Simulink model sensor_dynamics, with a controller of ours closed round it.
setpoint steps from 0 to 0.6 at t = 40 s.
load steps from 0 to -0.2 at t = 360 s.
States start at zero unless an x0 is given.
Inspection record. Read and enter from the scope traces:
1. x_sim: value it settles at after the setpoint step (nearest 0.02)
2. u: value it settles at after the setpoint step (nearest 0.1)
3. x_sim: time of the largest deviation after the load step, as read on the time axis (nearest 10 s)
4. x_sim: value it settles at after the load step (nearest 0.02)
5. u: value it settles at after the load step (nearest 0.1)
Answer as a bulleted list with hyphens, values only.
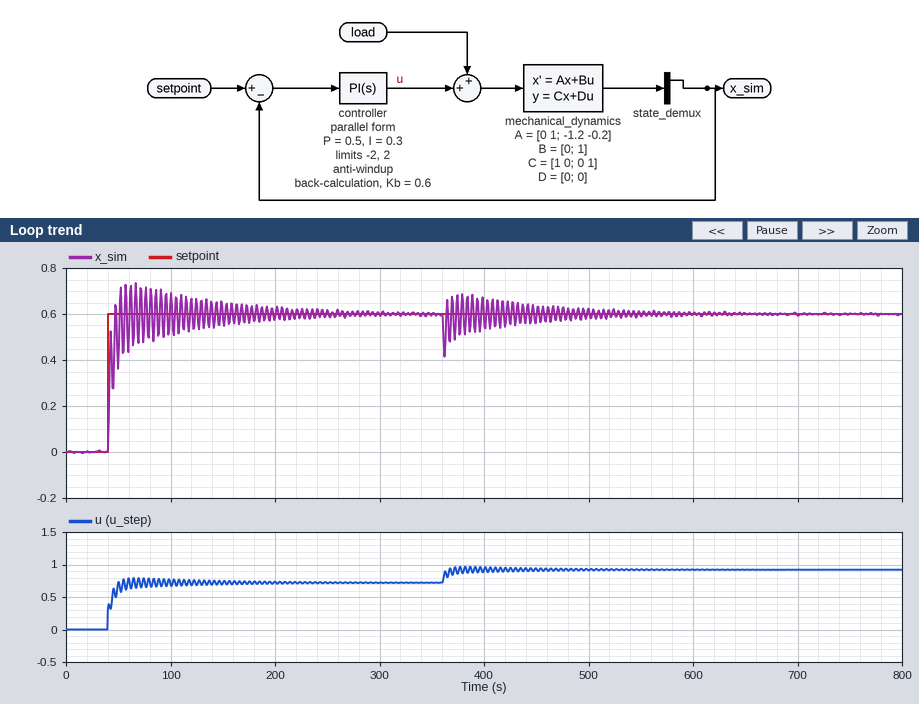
- 0.60
- 0.7
- 360 s
- 0.60
- 0.9
